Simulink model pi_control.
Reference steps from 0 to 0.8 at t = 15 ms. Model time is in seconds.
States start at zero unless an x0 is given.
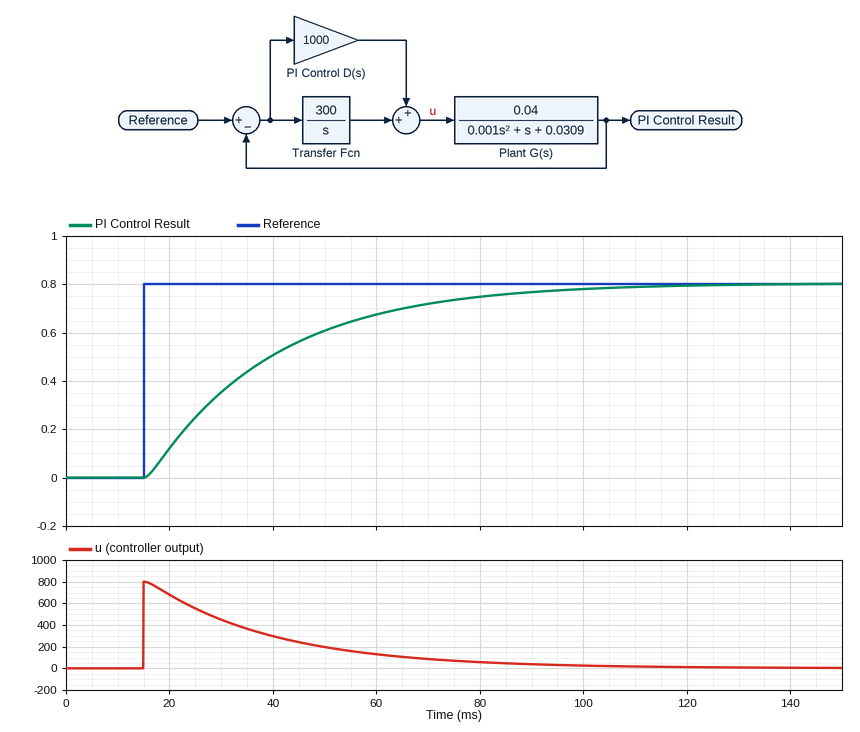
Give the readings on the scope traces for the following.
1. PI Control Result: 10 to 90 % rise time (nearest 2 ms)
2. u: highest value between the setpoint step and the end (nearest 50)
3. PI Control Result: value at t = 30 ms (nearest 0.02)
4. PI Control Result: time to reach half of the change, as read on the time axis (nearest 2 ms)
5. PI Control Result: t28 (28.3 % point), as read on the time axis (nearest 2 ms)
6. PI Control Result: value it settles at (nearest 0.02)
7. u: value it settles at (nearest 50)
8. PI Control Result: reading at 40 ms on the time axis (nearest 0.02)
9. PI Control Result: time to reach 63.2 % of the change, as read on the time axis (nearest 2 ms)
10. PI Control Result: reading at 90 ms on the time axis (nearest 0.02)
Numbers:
52 ms
800
0.36
32 ms
24 ms
0.80
0
0.50
40 ms
0.76
